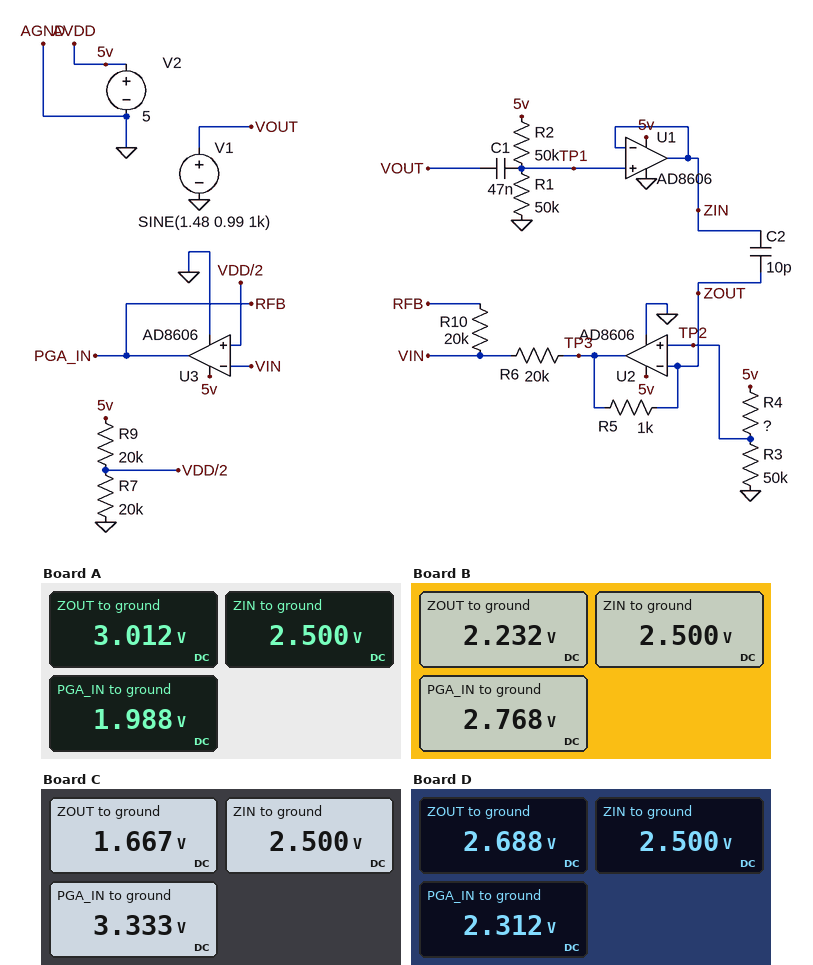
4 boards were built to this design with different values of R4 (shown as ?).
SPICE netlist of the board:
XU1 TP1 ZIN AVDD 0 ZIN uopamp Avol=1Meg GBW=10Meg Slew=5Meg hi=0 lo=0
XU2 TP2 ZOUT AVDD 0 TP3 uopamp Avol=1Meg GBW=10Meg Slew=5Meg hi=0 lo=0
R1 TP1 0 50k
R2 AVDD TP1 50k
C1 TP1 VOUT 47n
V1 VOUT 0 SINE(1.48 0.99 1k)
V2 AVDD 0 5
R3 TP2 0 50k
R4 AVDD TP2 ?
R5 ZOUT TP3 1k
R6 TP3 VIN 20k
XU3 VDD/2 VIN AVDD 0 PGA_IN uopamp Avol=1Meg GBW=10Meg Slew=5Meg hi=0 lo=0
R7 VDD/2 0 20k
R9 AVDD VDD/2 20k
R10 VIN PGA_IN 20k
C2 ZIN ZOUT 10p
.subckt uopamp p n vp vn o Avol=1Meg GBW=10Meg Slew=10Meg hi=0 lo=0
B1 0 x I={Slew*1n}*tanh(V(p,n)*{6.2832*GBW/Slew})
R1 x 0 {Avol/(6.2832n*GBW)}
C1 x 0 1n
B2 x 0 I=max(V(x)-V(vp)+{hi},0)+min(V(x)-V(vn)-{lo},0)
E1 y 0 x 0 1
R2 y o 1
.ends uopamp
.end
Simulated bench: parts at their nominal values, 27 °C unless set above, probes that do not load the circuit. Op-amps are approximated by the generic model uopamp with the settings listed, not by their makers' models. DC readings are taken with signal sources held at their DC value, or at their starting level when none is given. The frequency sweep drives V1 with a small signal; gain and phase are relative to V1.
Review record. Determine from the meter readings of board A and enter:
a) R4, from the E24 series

33 kΩ
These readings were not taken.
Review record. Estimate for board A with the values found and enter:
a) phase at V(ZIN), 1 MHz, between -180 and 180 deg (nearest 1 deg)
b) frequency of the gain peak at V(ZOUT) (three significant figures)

-6 deg
14.4 MHz
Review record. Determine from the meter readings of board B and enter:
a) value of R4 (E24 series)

62 kΩ
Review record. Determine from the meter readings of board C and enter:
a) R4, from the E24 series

100 kΩ
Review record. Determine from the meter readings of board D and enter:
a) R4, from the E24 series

43 kΩ
